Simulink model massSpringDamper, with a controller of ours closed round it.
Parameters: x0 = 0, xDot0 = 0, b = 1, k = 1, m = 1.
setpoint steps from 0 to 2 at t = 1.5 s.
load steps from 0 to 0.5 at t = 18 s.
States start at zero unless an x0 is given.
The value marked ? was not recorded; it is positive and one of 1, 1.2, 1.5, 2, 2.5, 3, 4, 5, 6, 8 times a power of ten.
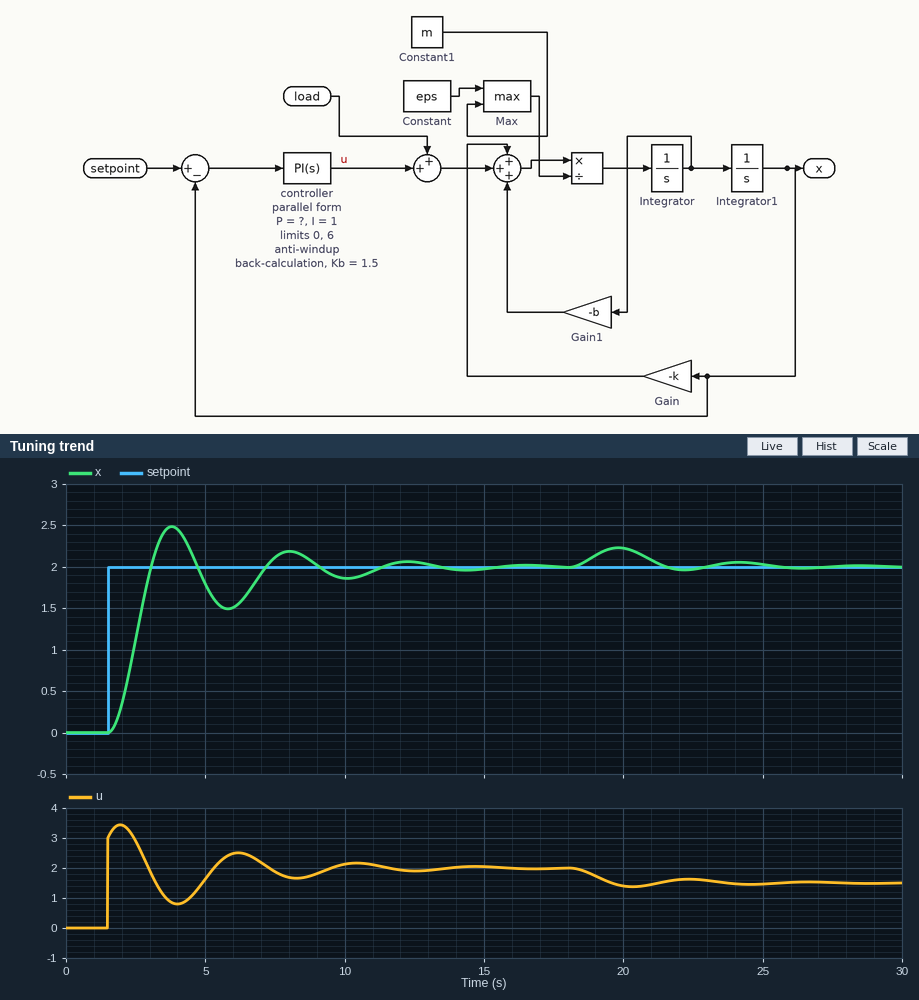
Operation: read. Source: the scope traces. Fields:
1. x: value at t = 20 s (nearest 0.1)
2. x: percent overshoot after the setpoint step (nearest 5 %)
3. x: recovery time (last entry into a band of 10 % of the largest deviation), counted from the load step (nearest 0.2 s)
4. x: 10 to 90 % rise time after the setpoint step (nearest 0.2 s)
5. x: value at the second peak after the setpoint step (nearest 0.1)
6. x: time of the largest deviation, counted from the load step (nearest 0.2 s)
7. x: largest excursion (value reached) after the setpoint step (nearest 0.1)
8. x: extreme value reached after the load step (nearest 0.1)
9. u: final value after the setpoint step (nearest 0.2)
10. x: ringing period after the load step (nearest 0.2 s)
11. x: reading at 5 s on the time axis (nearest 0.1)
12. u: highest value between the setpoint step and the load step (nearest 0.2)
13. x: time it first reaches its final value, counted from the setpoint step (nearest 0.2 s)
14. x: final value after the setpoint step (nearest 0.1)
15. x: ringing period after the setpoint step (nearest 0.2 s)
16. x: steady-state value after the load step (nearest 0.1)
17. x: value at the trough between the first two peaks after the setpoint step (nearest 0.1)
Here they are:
2.2
25 %
7.2 s
1.0 s
2.2
1.8 s
2.5
2.2
2.0
4.4 s
1.8
3.4
1.6 s
2.0
4.2 s
2.0
1.5
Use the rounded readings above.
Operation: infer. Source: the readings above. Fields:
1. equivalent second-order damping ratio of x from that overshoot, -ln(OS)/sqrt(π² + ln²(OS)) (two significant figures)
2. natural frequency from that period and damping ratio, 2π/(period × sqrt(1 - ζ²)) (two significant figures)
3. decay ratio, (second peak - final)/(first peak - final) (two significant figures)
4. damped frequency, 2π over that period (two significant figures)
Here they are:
0.40
1.6 rad/s
0.40
1.5 rad/s
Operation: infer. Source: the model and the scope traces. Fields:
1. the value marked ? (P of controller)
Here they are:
1.5
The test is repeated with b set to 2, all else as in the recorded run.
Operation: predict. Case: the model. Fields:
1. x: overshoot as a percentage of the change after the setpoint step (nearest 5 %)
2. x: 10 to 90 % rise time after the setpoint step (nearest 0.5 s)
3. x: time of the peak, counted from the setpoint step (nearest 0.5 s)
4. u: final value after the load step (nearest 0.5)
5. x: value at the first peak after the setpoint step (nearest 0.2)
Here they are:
10 %
1.5 s
3.0 s
1.5
2.2
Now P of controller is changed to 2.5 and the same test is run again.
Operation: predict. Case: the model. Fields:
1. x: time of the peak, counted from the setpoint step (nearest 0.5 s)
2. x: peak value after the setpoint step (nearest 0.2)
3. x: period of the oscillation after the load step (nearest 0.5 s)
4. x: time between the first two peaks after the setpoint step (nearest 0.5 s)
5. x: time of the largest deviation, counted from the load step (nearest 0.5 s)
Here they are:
2.0 s
2.6
3.5 s
3.5 s
1.5 s
